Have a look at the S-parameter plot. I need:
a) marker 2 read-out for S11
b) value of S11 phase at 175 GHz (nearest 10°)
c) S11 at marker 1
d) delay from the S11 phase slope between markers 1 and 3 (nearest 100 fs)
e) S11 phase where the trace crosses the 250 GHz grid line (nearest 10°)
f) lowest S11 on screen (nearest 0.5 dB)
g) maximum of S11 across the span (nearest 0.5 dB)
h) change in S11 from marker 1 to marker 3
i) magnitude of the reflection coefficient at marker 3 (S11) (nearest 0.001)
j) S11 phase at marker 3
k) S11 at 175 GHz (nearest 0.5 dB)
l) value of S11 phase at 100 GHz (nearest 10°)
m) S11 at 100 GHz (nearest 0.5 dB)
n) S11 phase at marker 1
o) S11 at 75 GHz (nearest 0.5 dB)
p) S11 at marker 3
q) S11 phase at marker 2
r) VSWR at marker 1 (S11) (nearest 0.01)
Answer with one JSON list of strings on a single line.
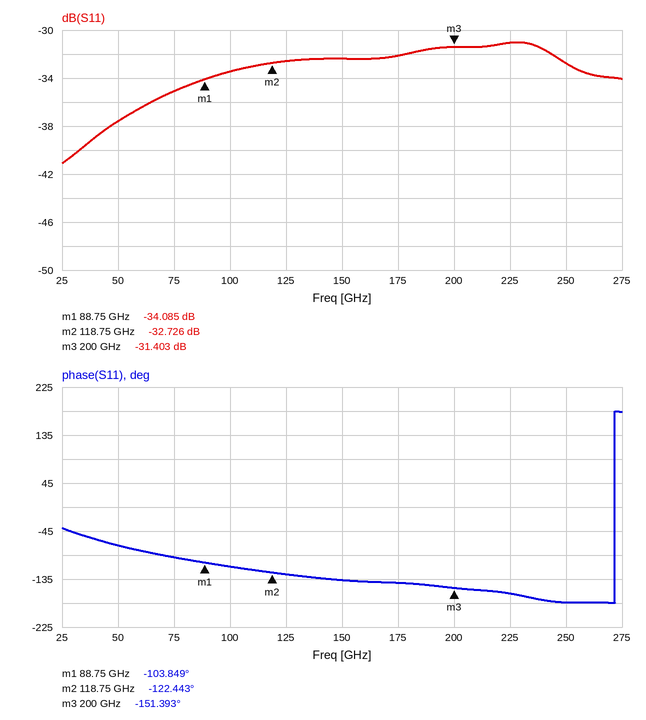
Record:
["-32.726 dB", "-140°", "-34.085 dB", "1.2 ps", "-180°", "-41.0 dB", "-31.0 dB", "2.682 dB", "0.027", "-151.393°", "-32.0 dB", "-110°", "-33.5 dB", "-103.849°", "-35.0 dB", "-31.403 dB", "-122.443°", "1.04"]
